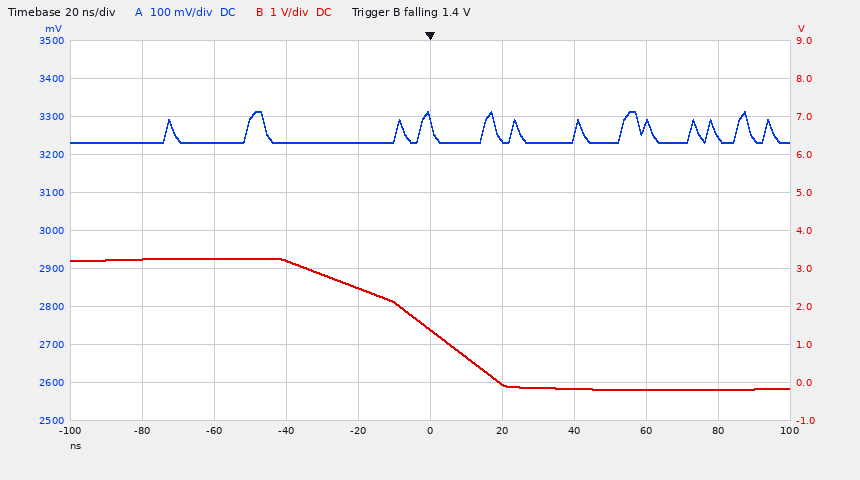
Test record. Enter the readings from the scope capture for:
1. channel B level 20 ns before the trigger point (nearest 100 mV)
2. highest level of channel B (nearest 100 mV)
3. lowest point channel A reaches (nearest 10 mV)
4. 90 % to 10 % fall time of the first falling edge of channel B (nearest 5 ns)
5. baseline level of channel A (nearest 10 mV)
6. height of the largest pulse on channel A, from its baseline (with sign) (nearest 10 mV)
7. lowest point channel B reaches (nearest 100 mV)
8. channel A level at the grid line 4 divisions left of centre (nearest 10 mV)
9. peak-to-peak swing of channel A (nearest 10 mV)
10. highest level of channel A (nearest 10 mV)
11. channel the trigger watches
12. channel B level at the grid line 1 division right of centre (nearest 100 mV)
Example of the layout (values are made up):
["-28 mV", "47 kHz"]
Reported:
["2.5 V", "3.3 V", "3.23 V", "50 ns", "3.23 V", "+80 mV", "-200 mV", "3.23 V", "80 mV", "3.31 V", "channel B", "0.0 V"]
